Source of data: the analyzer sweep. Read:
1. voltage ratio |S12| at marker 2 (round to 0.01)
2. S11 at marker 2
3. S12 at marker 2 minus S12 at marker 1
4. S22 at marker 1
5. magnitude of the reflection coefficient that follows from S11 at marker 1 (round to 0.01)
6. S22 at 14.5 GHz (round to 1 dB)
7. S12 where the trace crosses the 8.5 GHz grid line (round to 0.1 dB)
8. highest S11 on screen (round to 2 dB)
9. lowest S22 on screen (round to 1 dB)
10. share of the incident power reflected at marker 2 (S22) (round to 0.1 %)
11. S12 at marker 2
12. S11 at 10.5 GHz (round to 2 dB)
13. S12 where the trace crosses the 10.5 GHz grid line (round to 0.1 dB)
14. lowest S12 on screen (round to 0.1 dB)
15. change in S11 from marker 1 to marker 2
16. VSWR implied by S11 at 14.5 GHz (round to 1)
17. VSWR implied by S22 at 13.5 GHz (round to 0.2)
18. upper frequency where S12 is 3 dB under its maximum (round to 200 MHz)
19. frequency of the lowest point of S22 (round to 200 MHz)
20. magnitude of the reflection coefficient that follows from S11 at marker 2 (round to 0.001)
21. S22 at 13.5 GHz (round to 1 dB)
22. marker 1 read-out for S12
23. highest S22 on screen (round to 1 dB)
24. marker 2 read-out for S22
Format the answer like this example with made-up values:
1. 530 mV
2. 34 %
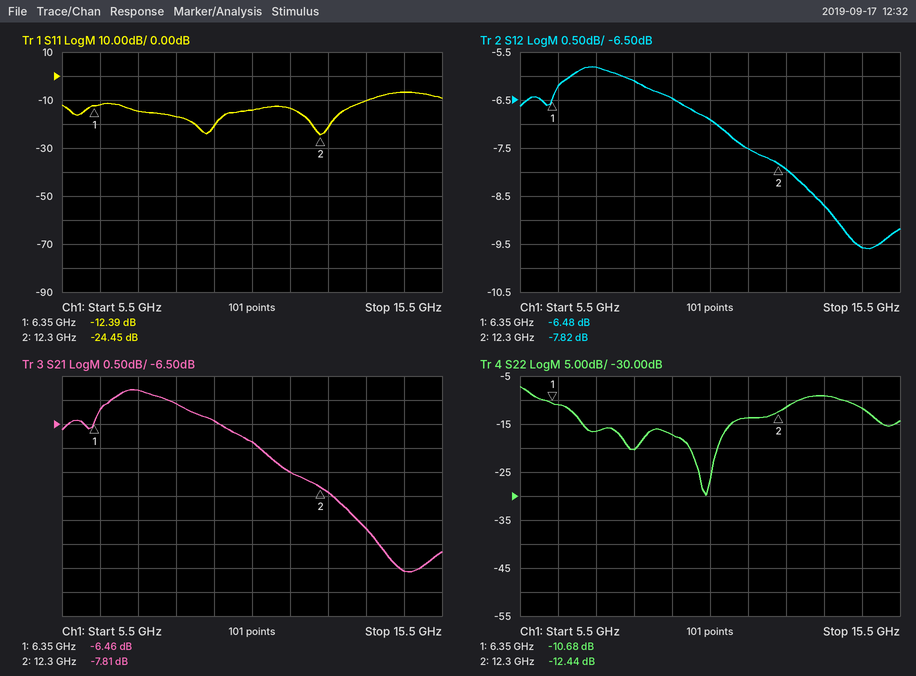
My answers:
1. 0.41
2. -24.45 dB
3. -1.34 dB
4. -10.68 dB
5. 0.24
6. -12 dB
7. -6.1 dB
8. -6 dB
9. -30 dB
10. 5.7 %
11. -7.82 dB
12. -14 dB
13. -6.9 dB
14. -9.6 dB
15. -12.06 dB
16. 3
17. 2.0
18. 13.6 GHz
19. 10.4 GHz
20. 0.060
21. -9 dB
22. -6.48 dB
23. -7 dB
24. -12.44 dB
